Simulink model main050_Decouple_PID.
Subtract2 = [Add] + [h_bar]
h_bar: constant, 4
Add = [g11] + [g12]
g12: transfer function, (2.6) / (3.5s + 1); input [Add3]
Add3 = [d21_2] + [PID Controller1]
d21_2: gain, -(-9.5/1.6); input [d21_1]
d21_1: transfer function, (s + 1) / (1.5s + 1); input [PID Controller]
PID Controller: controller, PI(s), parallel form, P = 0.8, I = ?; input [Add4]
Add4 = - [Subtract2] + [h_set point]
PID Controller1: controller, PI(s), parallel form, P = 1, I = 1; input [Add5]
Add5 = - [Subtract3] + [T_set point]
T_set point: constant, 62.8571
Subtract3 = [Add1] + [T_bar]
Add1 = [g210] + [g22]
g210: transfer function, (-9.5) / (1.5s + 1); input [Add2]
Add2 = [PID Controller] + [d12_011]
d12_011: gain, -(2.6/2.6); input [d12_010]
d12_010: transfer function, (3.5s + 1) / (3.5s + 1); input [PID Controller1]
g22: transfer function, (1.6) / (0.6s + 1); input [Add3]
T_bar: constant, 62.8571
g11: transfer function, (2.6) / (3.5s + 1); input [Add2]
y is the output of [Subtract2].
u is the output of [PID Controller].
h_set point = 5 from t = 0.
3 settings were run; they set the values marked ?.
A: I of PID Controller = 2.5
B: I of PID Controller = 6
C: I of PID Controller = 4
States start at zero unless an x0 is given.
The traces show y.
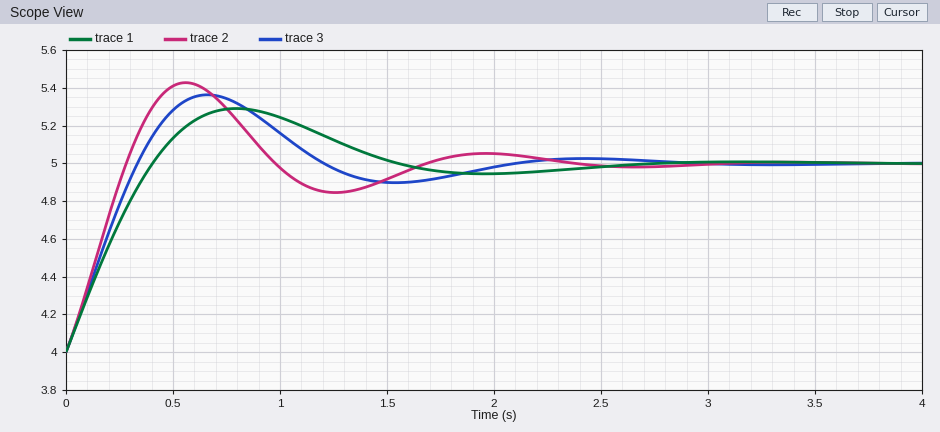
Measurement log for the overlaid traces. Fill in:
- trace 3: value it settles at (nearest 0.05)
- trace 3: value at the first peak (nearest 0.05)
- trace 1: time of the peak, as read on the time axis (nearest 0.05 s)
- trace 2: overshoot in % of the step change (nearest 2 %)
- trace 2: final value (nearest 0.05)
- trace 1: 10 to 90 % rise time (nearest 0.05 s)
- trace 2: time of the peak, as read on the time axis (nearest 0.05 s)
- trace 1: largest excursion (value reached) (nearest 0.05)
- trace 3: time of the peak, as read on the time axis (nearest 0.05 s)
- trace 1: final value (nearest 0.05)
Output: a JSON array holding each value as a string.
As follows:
["5.00", "5.35", "0.80 s", "42 %", "5.00", "0.30 s", "0.55 s", "5.30", "0.65 s", "5.00"]
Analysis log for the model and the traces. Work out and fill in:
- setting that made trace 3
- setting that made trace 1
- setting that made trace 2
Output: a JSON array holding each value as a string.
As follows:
["C", "A", "B"]
